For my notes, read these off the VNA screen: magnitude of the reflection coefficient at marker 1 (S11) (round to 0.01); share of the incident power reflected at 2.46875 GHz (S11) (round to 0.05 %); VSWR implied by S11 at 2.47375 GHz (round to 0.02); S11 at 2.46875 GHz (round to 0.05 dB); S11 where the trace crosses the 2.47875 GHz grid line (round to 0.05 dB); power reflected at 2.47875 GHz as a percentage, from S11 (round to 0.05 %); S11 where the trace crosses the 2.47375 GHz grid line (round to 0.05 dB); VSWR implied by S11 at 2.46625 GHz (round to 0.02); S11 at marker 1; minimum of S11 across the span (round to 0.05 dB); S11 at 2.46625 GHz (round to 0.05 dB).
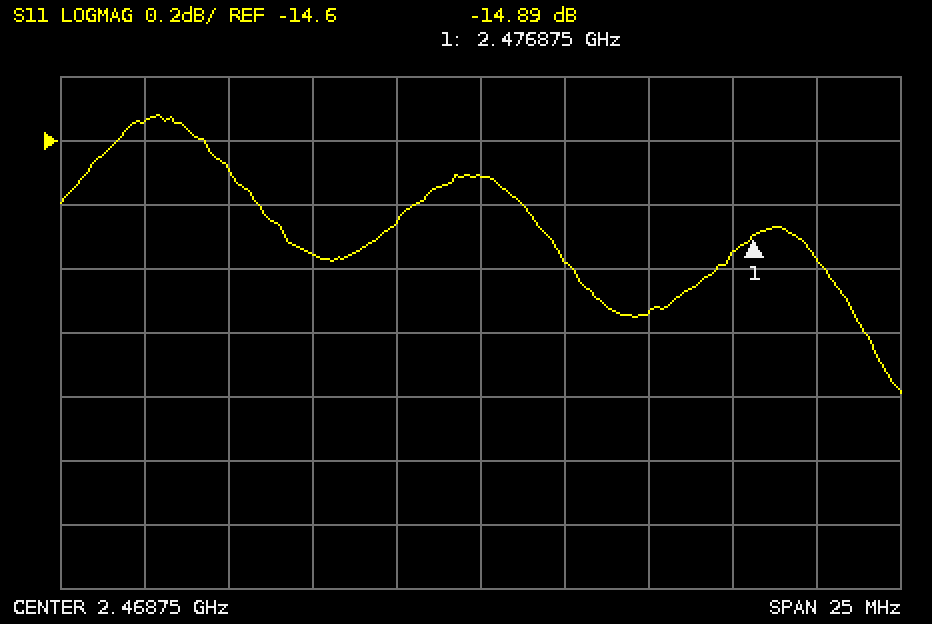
0.18
3.40 %
1.42
-14.70 dB
-14.95 dB
3.20 %
-15.15 dB
1.44
-14.89 dB
-15.40 dB
-14.85 dB
